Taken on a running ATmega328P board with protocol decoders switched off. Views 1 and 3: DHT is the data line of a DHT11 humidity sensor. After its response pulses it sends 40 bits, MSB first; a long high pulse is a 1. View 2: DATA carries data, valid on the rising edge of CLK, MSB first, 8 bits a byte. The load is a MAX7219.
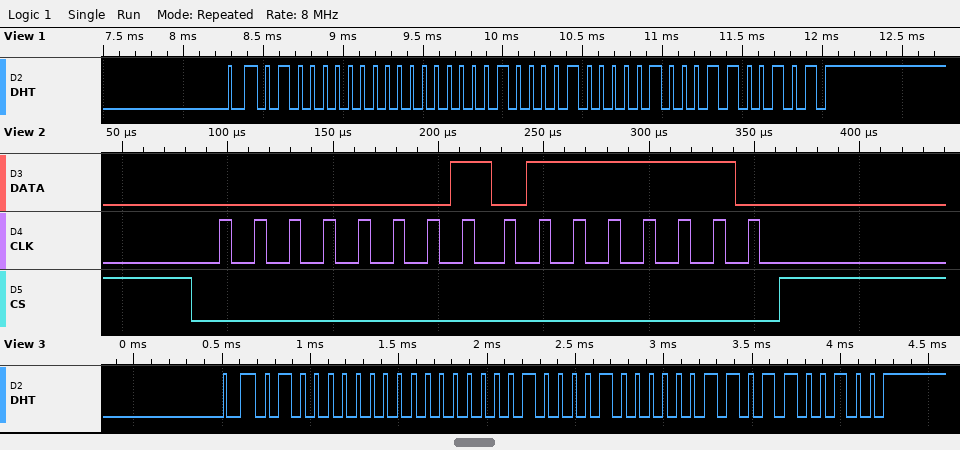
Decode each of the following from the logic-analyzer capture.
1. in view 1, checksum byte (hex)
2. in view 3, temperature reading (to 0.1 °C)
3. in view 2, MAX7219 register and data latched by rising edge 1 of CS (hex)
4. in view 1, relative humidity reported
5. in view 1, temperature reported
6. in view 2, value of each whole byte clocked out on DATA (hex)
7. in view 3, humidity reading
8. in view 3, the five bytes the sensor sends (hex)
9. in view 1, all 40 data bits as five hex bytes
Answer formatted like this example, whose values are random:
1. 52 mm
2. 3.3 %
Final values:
1. 0x65
2. 33.3 °C
3. register 0x1, data 0x7E
4. 64 %
5. 33.4 °C
6. 01 7E
7. 64 %
8. 40 00 21 03 64
9. 40 00 21 04 65
